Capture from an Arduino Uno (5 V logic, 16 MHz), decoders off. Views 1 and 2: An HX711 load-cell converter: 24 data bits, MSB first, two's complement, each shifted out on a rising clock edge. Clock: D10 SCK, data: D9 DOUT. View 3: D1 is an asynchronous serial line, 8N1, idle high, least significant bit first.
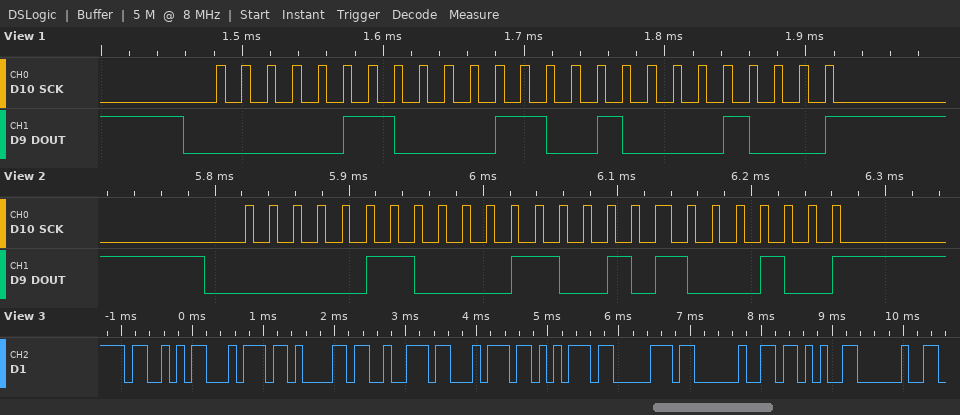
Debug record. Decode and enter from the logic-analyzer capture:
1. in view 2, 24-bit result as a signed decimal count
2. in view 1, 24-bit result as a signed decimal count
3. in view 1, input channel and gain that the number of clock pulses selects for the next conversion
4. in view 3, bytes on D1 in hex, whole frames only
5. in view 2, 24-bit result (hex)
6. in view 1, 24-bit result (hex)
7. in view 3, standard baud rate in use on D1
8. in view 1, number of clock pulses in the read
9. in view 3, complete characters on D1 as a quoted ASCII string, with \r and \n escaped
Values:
399684
399624
channel A, gain 128
0x53 0x74 0x61 0x72 0x74 0x75 0x70 0x20 0x2B 0x20
0x061944
0x061908
9600 baud
25
"Startup + "
